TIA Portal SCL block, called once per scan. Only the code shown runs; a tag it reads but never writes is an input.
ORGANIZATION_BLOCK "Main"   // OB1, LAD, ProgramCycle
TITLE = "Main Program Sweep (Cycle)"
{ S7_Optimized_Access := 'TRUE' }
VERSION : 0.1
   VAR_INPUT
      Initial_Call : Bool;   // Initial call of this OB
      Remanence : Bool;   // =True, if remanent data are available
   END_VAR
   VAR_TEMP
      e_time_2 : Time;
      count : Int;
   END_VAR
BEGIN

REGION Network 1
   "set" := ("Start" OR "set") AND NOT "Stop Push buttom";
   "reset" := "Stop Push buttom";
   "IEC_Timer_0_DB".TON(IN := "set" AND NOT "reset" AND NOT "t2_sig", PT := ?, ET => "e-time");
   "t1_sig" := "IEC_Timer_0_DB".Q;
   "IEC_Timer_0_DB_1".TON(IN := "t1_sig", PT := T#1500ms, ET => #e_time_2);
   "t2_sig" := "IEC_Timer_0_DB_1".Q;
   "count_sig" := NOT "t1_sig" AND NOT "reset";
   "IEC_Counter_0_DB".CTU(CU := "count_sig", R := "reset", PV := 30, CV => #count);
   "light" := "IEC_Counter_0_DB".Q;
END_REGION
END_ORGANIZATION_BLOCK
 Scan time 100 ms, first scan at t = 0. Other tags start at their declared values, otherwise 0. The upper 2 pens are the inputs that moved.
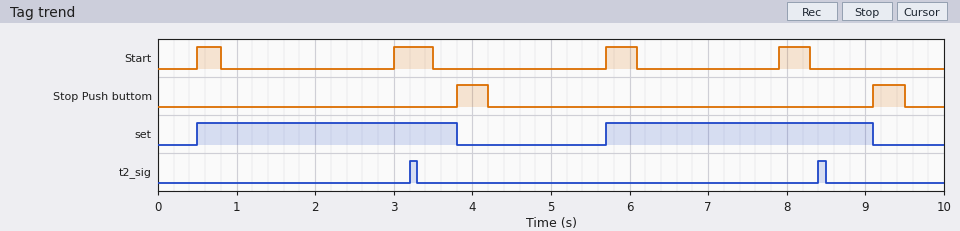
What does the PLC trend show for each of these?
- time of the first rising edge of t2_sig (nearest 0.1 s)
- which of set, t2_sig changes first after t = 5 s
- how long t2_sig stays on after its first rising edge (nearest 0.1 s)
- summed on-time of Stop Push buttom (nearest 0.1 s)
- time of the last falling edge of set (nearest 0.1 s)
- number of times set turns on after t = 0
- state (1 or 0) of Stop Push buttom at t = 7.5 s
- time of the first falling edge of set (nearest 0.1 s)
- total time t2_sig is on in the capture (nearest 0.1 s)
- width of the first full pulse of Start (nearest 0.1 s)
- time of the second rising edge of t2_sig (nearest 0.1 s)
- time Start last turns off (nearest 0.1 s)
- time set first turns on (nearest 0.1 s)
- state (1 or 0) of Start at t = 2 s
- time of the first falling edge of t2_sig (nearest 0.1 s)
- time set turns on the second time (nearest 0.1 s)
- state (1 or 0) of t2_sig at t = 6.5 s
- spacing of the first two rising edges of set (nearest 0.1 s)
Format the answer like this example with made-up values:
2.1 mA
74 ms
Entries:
3.2 s
set
0.1 s
0.8 s
9.1 s
2
0
3.8 s
0.2 s
0.3 s
8.4 s
8.3 s
0.5 s
0
3.3 s
5.7 s
0
5.2 s
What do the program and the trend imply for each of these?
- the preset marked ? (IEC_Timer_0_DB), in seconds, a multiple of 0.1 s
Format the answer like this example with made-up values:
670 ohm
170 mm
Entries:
1.2 s
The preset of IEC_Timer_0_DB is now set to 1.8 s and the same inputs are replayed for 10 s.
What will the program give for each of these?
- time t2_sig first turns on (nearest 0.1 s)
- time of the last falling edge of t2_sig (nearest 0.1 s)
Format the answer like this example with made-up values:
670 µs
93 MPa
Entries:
9.0 s
9.1 s
